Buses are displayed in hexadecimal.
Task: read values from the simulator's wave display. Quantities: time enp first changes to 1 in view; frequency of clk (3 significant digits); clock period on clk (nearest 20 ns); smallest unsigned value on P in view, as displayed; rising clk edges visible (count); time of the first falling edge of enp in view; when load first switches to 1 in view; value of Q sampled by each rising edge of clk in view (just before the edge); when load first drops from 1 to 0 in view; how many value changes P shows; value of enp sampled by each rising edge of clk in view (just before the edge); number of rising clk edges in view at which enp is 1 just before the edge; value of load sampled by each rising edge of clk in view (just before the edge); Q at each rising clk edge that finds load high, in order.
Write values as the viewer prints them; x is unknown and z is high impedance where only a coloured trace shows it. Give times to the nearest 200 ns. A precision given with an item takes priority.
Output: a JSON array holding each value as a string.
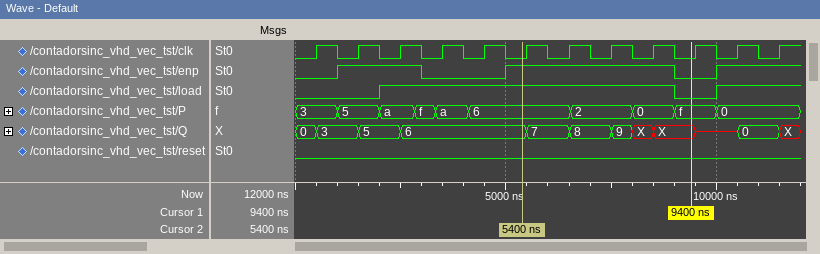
["1000 ns", "1.00 MHz", "1000 ns", "0", "12", "3000 ns", "2000 ns", "0, 3, 5, 6, 6, 6, 7, 8, X, X, x, 0", "9000 ns", "9", "0 1 1 0 0 1 1 1 1 0 1 1", "8", "0 0 1 1 1 1 1 1 1 0 1 1", "5, 6, 6, 6, 7, 8, X, x, 0"]
